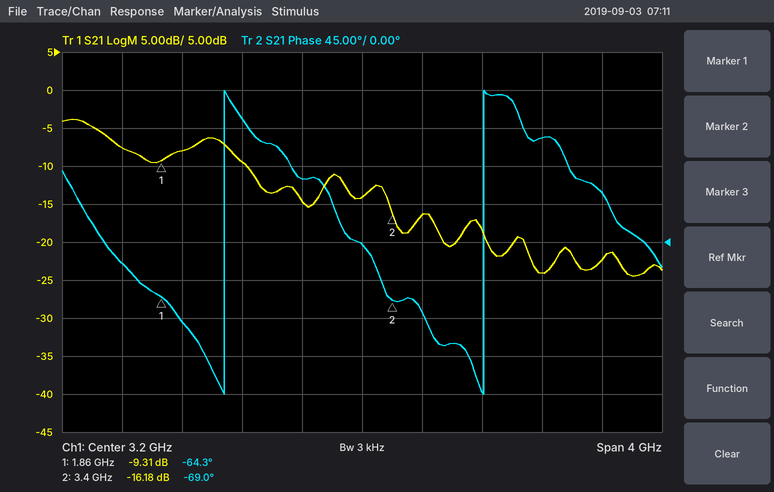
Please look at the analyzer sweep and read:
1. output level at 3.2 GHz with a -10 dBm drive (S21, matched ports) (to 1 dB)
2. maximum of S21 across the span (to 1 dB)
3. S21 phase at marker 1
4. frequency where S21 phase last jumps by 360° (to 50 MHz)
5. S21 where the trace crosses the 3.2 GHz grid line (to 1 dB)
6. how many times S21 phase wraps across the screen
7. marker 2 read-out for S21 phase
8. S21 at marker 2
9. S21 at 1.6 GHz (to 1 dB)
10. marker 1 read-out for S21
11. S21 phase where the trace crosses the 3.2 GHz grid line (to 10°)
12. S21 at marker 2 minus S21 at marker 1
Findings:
-24 dBm
-4 dB
-64.3°
4.00 GHz
-14 dB
2
-69.0°
-16.18 dB
-8 dB
-9.31 dB
0°
-6.87 dB
